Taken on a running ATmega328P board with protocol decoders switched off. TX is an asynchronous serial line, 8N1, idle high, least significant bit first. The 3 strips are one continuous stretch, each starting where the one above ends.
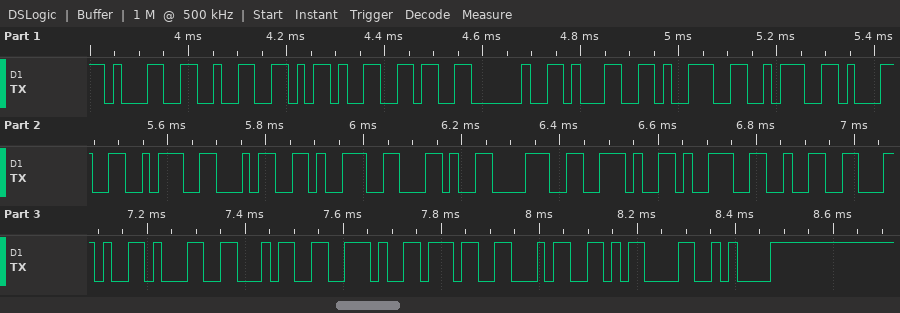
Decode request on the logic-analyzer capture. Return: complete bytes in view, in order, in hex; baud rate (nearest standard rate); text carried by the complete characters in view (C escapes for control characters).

0x31 0x32 0x2D 0x36 0x20 0x31 0x39 0x3A 0x31 0x3A 0x34 0x39 0x2C 0x38 0x2E 0x39 0x32 0x2C 0x31 0x34 0x2E 0x37 0x34 0x0D 0x0A
57600 baud
"12-6 19:1:49,8.92,14.74\r\n"
